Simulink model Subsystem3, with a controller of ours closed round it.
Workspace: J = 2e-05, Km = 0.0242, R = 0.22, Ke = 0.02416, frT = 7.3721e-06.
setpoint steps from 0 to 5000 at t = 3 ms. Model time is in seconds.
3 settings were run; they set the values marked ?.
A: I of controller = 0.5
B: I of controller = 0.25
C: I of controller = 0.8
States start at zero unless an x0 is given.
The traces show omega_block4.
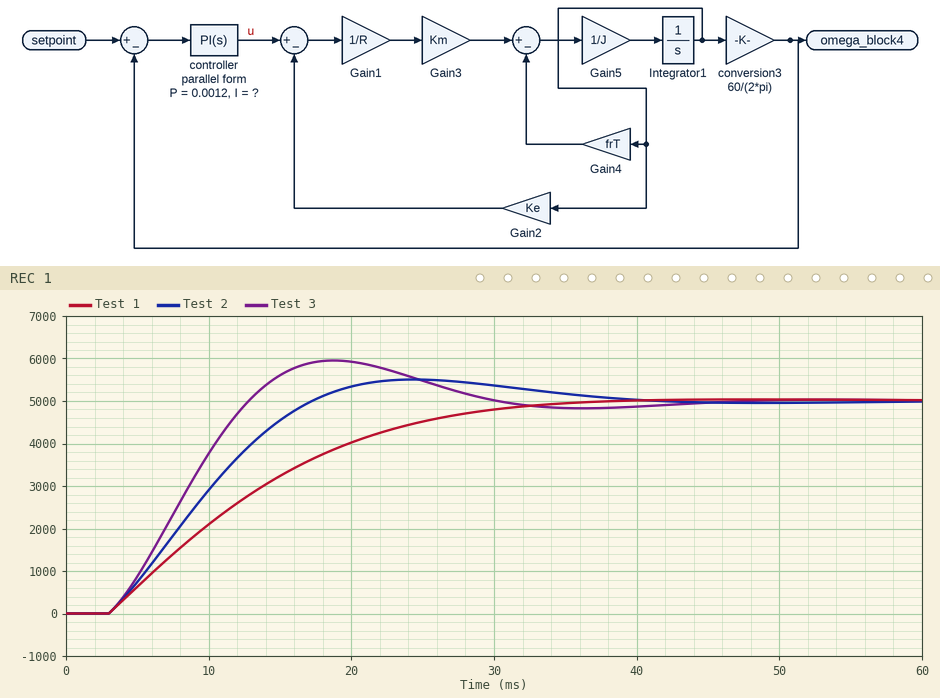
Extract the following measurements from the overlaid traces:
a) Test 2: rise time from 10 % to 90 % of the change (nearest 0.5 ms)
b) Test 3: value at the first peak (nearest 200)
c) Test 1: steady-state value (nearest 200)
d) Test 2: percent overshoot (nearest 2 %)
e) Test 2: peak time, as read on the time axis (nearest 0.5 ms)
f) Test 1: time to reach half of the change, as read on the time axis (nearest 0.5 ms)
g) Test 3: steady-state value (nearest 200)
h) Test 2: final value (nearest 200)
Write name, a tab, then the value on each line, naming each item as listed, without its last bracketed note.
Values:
Test 2: rise time from 10 % to 90 % of the change	10.5 ms
Test 3: value at the first peak	6000
Test 1: steady-state value	5000
Test 2: percent overshoot	10 %
Test 2: peak time, as read on the time axis	24.5 ms
Test 1: time to reach half of the change, as read on the time axis	11.5 ms
Test 3: steady-state value	5000
Test 2: final value	5000
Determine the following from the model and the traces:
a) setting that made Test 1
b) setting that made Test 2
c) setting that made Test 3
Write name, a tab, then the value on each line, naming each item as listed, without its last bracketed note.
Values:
setting that made Test 1	B
setting that made Test 2	A
setting that made Test 3	C
